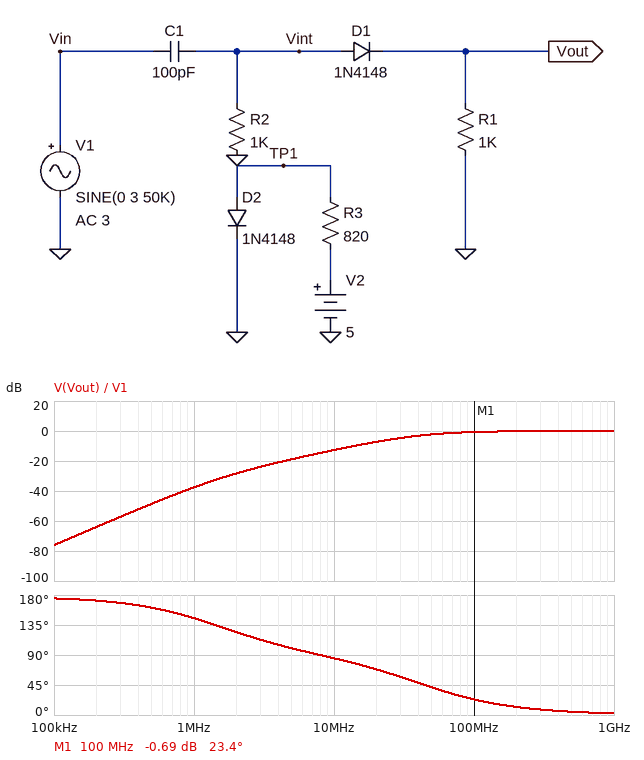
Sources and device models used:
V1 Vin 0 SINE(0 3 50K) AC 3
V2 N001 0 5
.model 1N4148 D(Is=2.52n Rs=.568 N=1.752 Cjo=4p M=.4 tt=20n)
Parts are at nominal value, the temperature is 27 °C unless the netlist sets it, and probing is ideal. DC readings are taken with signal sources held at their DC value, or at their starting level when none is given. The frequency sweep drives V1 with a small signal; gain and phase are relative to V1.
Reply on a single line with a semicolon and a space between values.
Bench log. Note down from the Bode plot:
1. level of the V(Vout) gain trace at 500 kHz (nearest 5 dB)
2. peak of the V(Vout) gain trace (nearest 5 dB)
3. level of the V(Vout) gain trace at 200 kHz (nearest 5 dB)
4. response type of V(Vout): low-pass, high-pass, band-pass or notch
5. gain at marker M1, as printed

-50 dB; 0 dB; -65 dB; high-pass; -0.69 dB
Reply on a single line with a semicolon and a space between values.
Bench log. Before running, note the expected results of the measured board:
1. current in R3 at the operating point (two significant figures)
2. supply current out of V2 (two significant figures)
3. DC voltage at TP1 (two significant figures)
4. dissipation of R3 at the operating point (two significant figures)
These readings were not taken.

5.3 mA; 5.3 mA; 660 mV; 23 mW
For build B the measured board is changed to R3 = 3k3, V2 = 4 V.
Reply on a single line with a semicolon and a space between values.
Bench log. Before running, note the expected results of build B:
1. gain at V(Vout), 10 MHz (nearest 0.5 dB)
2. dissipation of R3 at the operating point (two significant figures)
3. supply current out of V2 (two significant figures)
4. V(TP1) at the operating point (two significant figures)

-12.5 dB; 3.5 mW; 1.0 mA; 590 mV
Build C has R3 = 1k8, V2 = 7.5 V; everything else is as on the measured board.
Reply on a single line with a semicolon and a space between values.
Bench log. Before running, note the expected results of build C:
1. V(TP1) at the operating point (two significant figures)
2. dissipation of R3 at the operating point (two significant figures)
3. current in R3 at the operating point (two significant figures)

650 mV; 26 mW; 3.8 mA
